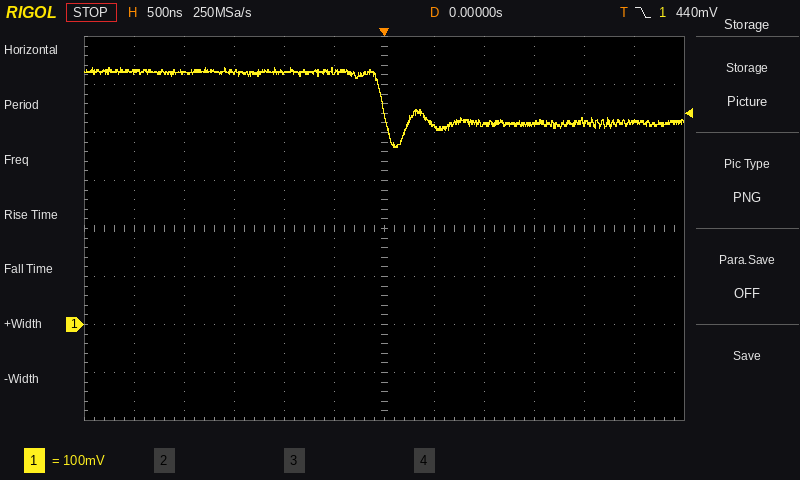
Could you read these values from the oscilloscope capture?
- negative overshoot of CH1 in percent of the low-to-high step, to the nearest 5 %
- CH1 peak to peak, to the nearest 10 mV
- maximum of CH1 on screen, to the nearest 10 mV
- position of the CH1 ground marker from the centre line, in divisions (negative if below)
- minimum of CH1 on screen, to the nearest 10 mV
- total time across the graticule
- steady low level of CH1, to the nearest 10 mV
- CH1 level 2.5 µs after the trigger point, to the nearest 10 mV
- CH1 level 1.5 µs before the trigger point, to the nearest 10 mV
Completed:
45 %
170 mV
540 mV
-2.0 div
370 mV
6 µs
420 mV
420 mV
530 mV
